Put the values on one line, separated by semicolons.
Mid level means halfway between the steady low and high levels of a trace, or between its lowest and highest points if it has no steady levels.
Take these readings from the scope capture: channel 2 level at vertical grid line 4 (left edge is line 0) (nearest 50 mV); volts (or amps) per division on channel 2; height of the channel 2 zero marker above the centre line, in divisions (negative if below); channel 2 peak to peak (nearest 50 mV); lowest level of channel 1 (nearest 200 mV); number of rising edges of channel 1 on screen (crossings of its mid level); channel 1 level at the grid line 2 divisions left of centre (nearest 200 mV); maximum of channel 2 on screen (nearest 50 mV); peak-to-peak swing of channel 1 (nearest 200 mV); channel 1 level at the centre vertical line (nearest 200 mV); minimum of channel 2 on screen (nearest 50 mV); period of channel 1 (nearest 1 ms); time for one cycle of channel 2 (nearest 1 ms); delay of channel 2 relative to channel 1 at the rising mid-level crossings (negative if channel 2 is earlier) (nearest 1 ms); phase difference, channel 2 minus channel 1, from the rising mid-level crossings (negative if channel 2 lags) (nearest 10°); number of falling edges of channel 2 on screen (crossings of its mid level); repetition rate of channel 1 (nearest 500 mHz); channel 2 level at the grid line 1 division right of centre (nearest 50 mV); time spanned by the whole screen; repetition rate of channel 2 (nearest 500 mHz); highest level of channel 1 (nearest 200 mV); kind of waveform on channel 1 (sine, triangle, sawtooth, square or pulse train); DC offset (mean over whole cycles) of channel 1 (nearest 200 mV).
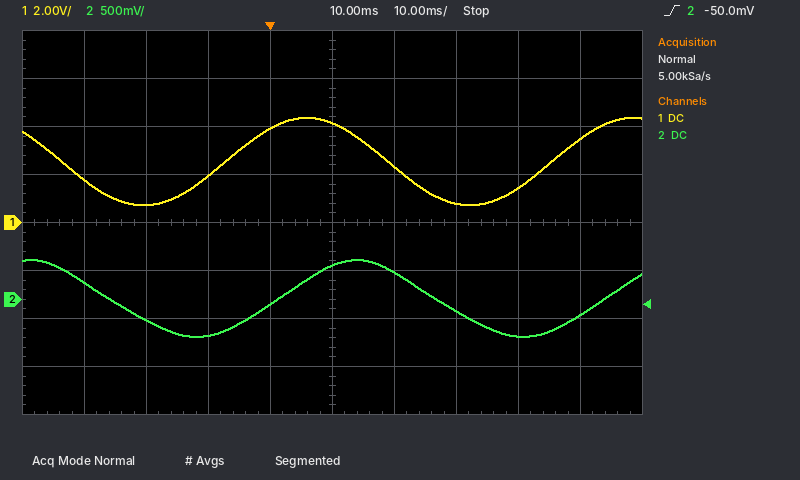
-50 mV; 500 mV; -1.6 div; 800 mV; 800 mV; 2; 2.0 V; 400 mV; 3.6 V; 4.2 V; -400 mV; 53 ms; 53 ms; +9 ms; -60°; 2; 19.0 Hz; 300 mV; 100 ms; 19.0 Hz; 4.4 V; sine; 2.6 V
